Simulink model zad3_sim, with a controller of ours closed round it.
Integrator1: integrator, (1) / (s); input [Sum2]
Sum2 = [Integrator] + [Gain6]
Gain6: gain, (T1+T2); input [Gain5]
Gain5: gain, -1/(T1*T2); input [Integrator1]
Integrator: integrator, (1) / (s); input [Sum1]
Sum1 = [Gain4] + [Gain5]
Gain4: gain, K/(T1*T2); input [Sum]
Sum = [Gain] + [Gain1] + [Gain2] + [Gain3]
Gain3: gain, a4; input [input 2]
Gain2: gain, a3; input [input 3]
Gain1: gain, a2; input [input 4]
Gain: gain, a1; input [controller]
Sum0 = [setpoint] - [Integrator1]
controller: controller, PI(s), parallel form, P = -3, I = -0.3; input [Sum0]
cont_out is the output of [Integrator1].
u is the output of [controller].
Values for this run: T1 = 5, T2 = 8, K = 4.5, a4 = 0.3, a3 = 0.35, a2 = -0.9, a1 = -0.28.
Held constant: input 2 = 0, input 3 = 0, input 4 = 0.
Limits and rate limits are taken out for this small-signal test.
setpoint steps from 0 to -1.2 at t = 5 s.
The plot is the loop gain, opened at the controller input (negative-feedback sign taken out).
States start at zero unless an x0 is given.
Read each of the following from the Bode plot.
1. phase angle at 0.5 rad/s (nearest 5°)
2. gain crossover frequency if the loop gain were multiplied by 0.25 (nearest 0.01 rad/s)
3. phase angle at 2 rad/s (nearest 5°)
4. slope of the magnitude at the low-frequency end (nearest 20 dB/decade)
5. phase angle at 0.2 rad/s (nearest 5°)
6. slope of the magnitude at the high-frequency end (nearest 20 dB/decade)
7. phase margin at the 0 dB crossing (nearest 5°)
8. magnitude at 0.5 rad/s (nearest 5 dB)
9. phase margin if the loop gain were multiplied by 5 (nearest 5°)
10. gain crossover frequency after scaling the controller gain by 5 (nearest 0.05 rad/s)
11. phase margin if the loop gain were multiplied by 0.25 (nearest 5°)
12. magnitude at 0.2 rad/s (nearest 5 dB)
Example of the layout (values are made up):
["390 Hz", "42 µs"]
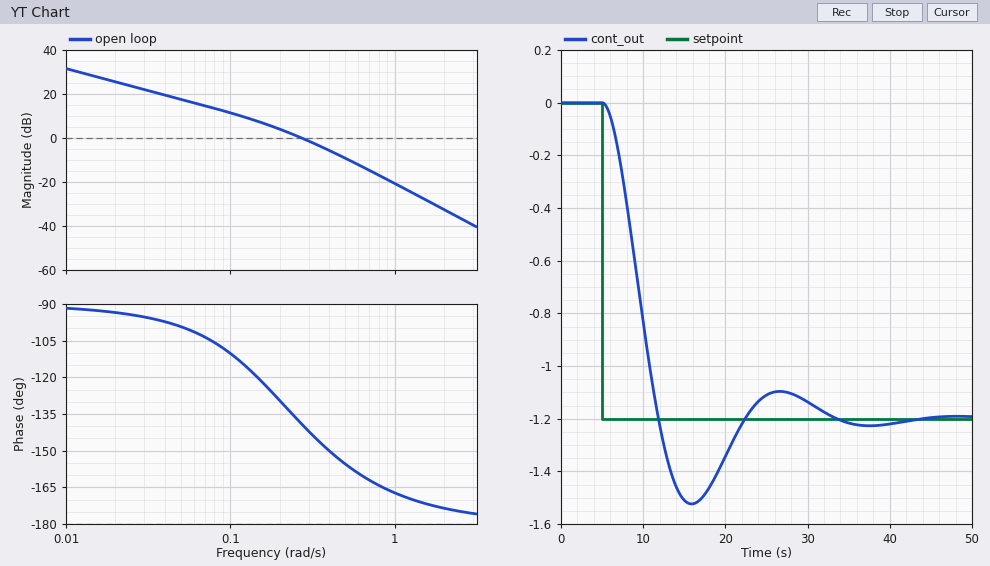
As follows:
["-155°", "0.09 rad/s", "-175°", "-20 dB/decade", "-130°", "-40 dB/decade", "40°", "-10 dB", "20°", "0.65 rad/s", "70°", "5 dB"]
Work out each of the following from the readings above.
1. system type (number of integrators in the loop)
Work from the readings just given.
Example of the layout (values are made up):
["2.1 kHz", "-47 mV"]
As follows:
["1"]
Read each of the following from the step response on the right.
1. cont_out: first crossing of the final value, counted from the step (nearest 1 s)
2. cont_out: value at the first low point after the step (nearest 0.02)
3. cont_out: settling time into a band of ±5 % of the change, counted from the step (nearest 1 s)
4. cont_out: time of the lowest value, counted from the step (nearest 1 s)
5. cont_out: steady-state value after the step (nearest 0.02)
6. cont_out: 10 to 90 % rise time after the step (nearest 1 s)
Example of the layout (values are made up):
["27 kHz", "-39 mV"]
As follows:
["7 s", "-1.52", "25 s", "11 s", "-1.20", "5 s"]
